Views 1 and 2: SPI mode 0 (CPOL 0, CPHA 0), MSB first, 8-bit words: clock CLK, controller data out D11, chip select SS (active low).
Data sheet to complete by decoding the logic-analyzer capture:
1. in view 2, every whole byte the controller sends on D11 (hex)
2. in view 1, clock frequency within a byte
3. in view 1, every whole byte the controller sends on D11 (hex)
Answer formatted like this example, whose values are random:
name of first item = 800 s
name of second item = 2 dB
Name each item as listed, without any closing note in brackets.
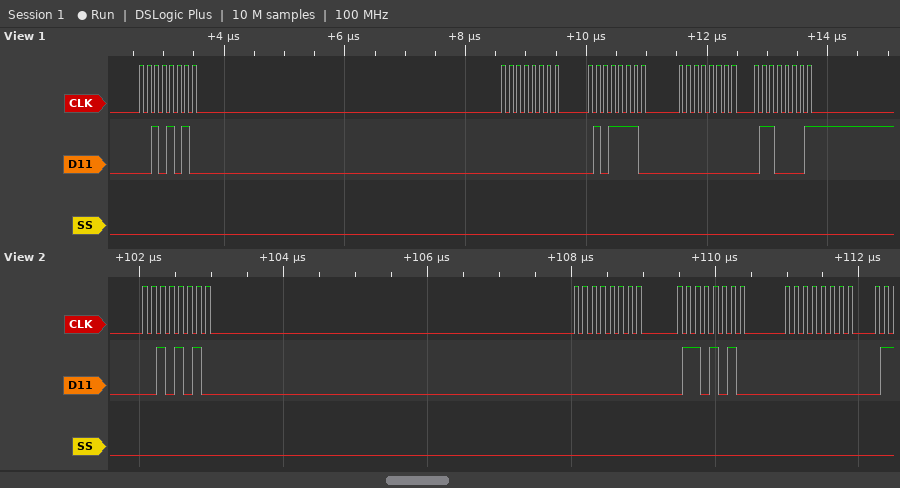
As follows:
in view 2, every whole byte the controller sends on D11 = 2A 00 6A 00
in view 1, clock frequency within a byte = 8 MHz
in view 1, every whole byte the controller sends on D11 = 2A 00 5E 00 61
